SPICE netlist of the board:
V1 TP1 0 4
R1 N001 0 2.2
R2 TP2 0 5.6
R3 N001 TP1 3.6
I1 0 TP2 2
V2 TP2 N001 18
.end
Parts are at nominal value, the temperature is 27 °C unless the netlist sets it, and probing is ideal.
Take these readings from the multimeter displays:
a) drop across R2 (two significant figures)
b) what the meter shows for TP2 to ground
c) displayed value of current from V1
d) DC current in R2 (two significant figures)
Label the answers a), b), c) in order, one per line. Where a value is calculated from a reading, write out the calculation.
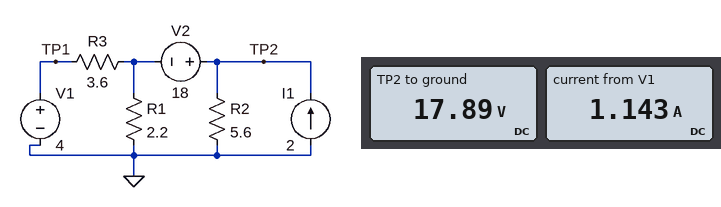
a) 17.89 V = 18 V
b) 17.89 V
c) 1.143 A
d) (17.89 V) / 5.6 Ω = 3.2 A
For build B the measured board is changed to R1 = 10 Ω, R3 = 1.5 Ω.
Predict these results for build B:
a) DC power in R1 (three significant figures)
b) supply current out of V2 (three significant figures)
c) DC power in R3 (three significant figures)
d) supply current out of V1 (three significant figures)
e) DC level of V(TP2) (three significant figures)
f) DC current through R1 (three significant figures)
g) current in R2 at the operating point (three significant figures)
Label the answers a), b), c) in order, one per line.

a) 236 mW
b) 1.49 A
c) 4.05 W
d) 1.64 A
e) 19.5 V
f) 154 mA
g) 3.49 A
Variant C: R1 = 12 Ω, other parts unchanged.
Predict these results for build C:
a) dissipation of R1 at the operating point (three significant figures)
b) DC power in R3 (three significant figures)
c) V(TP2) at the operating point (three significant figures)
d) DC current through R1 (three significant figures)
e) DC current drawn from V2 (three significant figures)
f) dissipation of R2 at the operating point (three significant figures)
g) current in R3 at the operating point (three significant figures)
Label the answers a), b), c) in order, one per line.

a) 3.05 mW
b) 4.88 W
c) 17.8 V
d) 15.9 mA
e) 1.18 A
f) 56.6 W
g) 1.16 A
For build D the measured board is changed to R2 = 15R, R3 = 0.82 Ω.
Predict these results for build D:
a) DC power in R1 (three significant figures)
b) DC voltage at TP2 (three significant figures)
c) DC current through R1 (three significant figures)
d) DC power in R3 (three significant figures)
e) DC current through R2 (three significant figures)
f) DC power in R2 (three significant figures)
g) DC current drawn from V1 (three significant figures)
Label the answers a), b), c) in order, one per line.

a) 4.84 W
b) 21.3 V
c) 1.48 A
d) 664 mW
e) 1.42 A
f) 30.1 W
g) 900 mA
